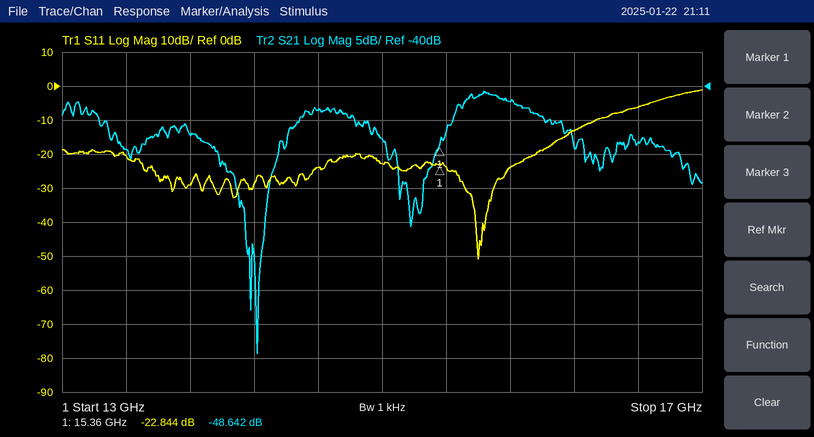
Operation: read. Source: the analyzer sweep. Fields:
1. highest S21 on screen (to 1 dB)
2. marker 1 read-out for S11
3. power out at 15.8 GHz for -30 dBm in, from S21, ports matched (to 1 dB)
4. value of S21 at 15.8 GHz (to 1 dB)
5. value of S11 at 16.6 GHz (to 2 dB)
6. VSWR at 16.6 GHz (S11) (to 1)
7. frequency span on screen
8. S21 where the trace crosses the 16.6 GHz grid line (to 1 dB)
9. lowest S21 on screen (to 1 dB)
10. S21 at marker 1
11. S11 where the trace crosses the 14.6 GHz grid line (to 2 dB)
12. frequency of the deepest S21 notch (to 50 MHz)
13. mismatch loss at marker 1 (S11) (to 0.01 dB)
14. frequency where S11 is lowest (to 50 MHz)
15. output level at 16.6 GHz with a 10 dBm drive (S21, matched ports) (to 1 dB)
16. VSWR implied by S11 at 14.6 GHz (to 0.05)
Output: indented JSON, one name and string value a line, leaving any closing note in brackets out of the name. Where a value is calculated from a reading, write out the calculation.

{
  "highest S21 on screen": "-41 dB",
  "marker 1 read-out for S11": "-22.844 dB",
  "power out at 15.8 GHz for -30 dBm in, from S21, ports matched": "-30 dBm + (-42 dB) = -72 dBm",
  "value of S21 at 15.8 GHz": "-42 dB",
  "value of S11 at 16.6 GHz": "-6 dB",
  "VSWR at 16.6 GHz (S11)": "|Γ| = 10^(-6/20) = 0.5012; VSWR = (1 + 0.5012)/(1 − 0.5012) ≈ 3",
  "frequency span on screen": "4 GHz",
  "S21 where the trace crosses the 16.6 GHz grid line": "-48 dB",
  "lowest S21 on screen": "-79 dB",
  "S21 at marker 1": "-48.642 dB",
  "S11 where the trace crosses the 14.6 GHz grid line": "-24 dB",
  "frequency of the deepest S21 notch": "14.20 GHz",
  "mismatch loss at marker 1 (S11)": "−10 log10(1 − 10^(-22.844/10)) ≈ 0.02 dB",
  "frequency where S11 is lowest": "15.60 GHz",
  "output level at 16.6 GHz with a 10 dBm drive (S21, matched ports)": "10 dBm + (-48 dB) = -38 dBm",
  "VSWR implied by S11 at 14.6 GHz": "|Γ| = 10^(-24/20) = 0.0631; VSWR = (1 + 0.0631)/(1 − 0.0631) ≈ 1.13, so 1.15 to the nearest 0.05"
}
